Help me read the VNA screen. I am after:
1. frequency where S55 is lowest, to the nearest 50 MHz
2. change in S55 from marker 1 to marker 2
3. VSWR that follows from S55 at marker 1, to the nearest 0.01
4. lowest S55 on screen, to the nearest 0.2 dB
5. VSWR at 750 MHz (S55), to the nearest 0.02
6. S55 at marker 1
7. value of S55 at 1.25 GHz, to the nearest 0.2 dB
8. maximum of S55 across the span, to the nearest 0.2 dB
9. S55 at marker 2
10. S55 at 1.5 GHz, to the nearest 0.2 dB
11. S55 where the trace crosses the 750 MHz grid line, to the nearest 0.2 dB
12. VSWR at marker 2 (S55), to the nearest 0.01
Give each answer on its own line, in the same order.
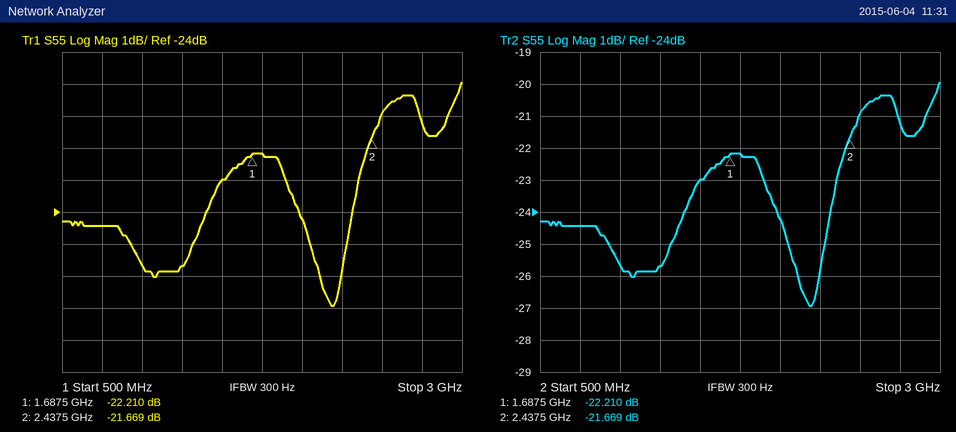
2.20 GHz
0.541 dB
1.17
-27.0 dB
1.12
-22.210 dB
-25.6 dB
-20.0 dB
-21.669 dB
-23.0 dB
-24.4 dB
1.18
